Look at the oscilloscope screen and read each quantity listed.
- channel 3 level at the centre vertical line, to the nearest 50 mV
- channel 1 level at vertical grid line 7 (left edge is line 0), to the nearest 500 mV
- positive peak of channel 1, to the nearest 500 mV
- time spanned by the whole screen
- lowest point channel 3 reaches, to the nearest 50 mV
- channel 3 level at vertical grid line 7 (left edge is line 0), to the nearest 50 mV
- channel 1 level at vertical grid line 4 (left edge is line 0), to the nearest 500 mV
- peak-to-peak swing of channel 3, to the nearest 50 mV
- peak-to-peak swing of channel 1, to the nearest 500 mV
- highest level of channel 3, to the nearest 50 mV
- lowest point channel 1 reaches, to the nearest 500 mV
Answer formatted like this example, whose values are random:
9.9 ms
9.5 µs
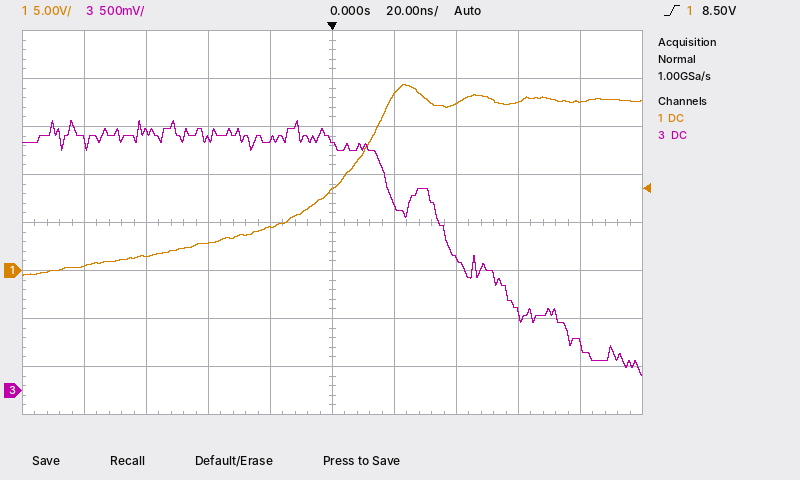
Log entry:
2.60 V
17.5 V
19.5 V
200 ns
150 mV
1.35 V
4.5 V
2.65 V
20.0 V
2.80 V
-500 mV
